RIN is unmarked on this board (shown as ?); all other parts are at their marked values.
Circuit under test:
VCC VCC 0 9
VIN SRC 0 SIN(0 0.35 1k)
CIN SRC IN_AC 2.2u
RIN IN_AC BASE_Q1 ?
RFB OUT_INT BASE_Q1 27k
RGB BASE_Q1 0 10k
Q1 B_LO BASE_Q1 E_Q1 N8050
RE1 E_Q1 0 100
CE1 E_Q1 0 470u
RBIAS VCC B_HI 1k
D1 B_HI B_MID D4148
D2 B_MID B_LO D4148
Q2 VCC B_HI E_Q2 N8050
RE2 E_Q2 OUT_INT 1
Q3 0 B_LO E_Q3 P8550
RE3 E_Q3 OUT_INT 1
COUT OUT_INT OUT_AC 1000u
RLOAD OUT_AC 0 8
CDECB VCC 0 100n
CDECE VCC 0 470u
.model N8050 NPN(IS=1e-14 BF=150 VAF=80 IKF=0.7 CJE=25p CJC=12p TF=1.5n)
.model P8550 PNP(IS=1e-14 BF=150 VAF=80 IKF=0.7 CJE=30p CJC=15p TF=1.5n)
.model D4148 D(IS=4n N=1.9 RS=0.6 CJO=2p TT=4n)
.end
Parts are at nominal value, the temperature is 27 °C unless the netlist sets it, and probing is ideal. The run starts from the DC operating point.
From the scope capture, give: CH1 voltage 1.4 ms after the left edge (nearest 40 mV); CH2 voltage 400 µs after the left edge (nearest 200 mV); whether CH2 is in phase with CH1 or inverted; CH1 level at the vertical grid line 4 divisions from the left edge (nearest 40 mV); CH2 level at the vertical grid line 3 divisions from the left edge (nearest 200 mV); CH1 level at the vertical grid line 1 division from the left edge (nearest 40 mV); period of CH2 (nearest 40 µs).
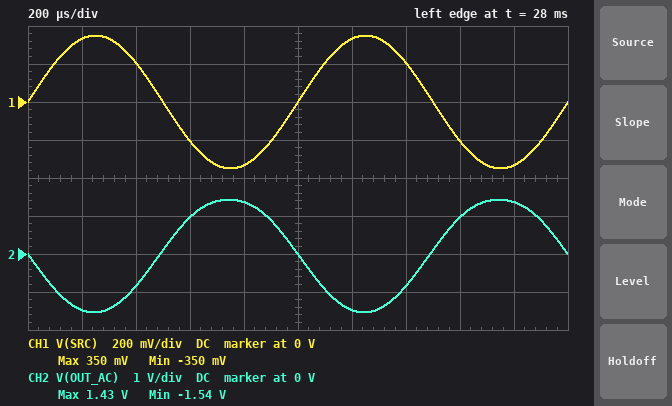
200 mV
-800 mV
inverted
-320 mV
1.0 V
320 mV
1.00 ms
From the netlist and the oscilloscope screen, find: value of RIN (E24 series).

3.9 kΩ
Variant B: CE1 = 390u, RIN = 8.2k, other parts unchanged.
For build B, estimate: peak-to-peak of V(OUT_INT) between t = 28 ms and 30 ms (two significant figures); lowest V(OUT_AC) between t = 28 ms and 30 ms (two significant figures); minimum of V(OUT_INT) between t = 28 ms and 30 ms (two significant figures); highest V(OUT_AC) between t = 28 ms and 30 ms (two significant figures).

1.5 V
-770 mV
3.8 V
760 mV
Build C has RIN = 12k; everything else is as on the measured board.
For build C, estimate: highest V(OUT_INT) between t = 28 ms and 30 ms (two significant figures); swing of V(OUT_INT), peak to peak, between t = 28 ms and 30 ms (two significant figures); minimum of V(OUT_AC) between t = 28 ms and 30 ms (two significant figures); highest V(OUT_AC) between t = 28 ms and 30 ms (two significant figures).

5.1 V
1.1 V
-530 mV
530 mV
